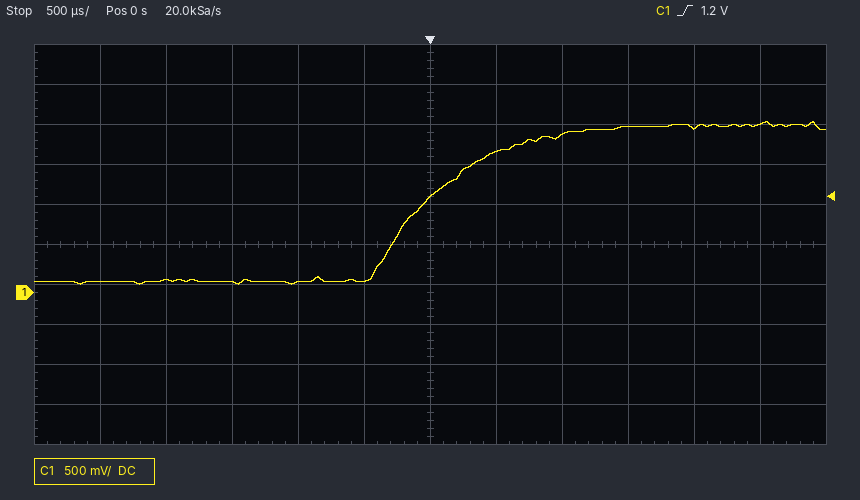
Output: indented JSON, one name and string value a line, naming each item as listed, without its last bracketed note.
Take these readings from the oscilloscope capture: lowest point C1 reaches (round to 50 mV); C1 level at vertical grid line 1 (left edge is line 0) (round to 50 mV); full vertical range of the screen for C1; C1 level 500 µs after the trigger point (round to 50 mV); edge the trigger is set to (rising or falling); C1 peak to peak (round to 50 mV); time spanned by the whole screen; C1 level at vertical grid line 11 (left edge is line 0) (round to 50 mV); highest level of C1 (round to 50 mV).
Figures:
{
  "lowest point C1 reaches": "100 mV",
  "C1 level at vertical grid line 1 (left edge is line 0)": "150 mV",
  "full vertical range of the screen for C1": "5 V",
  "C1 level 500 µs after the trigger point": "1.75 V",
  "edge the trigger is set to": "rising",
  "C1 peak to peak": "2.05 V",
  "time spanned by the whole screen": "6 ms",
  "C1 level at vertical grid line 11 (left edge is line 0)": "2.10 V",
  "highest level of C1": "2.15 V"
}
